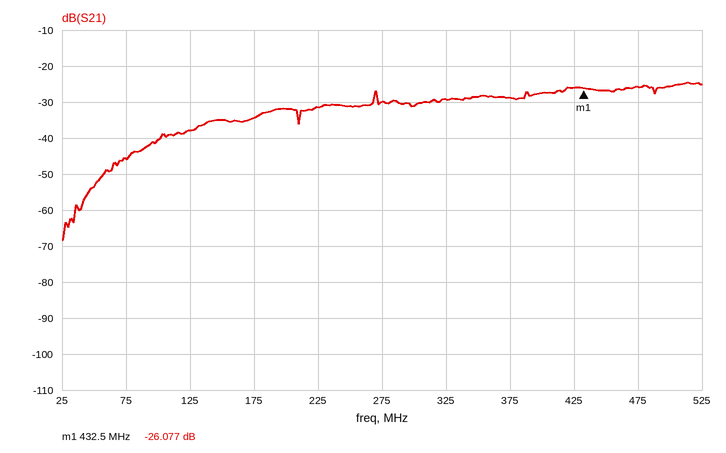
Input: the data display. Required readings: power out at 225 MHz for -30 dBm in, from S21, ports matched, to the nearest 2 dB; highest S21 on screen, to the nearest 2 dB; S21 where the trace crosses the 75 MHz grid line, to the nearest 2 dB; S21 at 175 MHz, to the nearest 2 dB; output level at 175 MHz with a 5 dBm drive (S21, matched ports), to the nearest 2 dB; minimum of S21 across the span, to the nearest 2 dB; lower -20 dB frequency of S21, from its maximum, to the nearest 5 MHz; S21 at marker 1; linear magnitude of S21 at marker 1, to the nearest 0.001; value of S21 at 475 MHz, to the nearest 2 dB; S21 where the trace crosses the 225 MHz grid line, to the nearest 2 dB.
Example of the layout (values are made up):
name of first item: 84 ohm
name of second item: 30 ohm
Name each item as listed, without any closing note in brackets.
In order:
power out at 225 MHz for -30 dBm in, from S21, ports matched, to the nearest 2 dB: -62 dBm
highest S21 on screen, to the nearest 2 dB: -24 dB
S21 where the trace crosses the 75 MHz grid line, to the nearest 2 dB: -46 dB
S21 at 175 MHz, to the nearest 2 dB: -34 dB
output level at 175 MHz with a 5 dBm drive (S21, matched ports), to the nearest 2 dB: -30 dBm
minimum of S21 across the span, to the nearest 2 dB: -68 dB
lower -20 dB frequency of S21, from its maximum, to the nearest 5 MHz: 80 MHz
S21 at marker 1: -26.077 dB
linear magnitude of S21 at marker 1, to the nearest 0.001: 0.050
value of S21 at 475 MHz, to the nearest 2 dB: -26 dB
S21 where the trace crosses the 225 MHz grid line, to the nearest 2 dB: -32 dB
